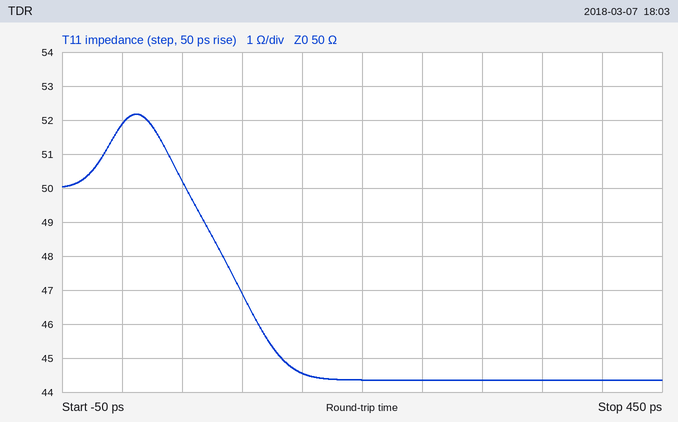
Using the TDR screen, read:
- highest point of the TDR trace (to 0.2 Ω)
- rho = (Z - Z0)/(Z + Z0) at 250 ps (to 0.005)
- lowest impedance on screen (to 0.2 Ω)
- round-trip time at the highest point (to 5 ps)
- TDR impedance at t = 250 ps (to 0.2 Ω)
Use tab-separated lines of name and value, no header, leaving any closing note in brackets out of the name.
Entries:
highest point of the TDR trace	52.2 Ω
rho = (Z - Z0)/(Z + Z0) at 250 ps	-0.060
lowest impedance on screen	44.4 Ω
round-trip time at the highest point	10 ps
TDR impedance at t = 250 ps	44.4 Ω
